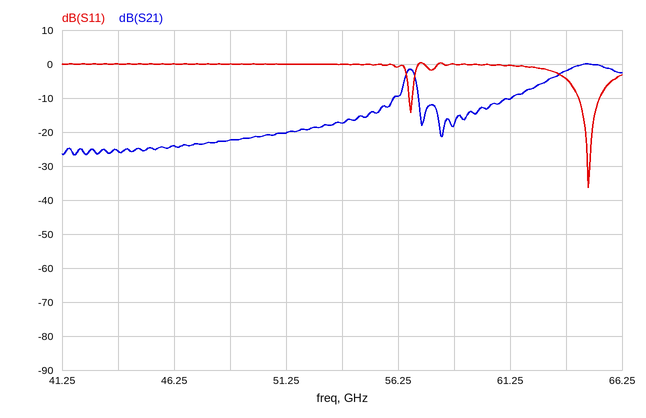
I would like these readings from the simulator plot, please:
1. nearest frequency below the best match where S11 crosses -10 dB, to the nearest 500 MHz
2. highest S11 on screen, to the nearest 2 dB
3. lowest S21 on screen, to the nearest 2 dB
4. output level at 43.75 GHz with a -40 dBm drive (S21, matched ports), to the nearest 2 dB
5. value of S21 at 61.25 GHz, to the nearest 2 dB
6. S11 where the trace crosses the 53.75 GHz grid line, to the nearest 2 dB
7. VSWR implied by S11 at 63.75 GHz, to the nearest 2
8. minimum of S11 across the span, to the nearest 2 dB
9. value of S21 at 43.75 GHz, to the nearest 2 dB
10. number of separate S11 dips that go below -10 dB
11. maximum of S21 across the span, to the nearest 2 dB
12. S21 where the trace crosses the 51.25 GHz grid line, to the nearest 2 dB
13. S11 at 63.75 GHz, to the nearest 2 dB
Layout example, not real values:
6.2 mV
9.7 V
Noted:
64.5 GHz
0 dB
-26 dB
-66 dBm
-10 dB
0 dB
4
-36 dB
-26 dB
2
0 dB
-20 dB
-4 dB
